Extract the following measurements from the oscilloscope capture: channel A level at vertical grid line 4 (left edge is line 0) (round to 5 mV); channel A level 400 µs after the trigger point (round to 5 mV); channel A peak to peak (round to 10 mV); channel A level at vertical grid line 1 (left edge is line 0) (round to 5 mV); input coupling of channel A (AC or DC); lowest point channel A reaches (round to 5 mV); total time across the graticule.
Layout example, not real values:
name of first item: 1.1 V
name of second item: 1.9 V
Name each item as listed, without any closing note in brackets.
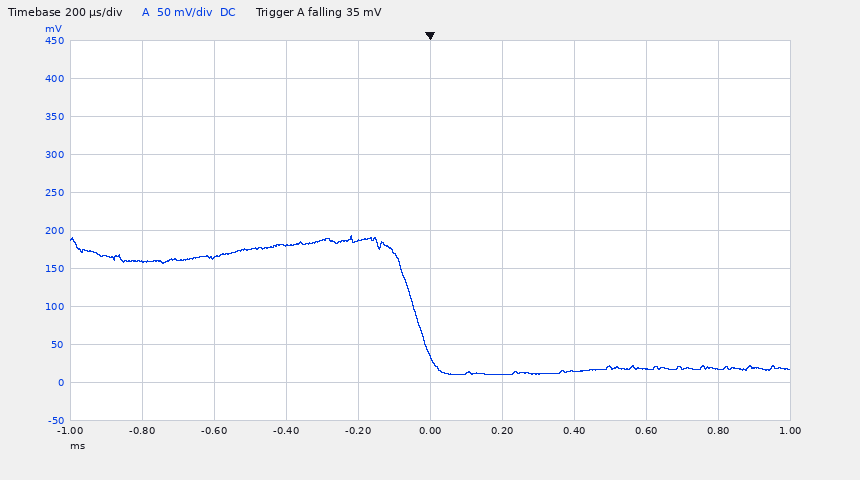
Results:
channel A level at vertical grid line 4 (left edge is line 0): 185 mV
channel A level 400 µs after the trigger point: 15 mV
channel A peak to peak: 180 mV
channel A level at vertical grid line 1 (left edge is line 0): 160 mV
input coupling of channel A: DC
lowest point channel A reaches: 10 mV
total time across the graticule: 2 ms
